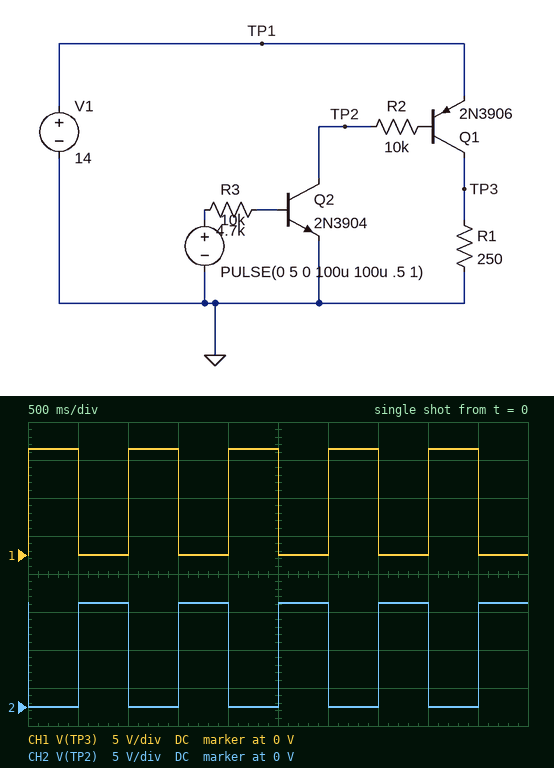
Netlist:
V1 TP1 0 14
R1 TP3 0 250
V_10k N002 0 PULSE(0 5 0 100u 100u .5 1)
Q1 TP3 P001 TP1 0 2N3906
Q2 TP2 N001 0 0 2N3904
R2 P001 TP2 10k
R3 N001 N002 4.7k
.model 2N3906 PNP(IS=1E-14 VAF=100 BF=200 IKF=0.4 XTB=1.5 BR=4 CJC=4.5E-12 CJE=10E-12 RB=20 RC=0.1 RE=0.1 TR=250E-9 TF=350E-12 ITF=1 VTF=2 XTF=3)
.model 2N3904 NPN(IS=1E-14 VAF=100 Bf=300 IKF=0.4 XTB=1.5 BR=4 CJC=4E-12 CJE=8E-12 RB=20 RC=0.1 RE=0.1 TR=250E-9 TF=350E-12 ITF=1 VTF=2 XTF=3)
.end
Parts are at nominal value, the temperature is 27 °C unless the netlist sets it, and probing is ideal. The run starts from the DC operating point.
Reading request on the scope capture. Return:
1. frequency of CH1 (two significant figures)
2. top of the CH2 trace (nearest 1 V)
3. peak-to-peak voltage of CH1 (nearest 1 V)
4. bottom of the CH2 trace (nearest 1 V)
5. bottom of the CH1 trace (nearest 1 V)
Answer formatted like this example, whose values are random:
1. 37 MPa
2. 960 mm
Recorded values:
1. 1.0 Hz
2. 14 V
3. 14 V
4. 0 V
5. 0 V
